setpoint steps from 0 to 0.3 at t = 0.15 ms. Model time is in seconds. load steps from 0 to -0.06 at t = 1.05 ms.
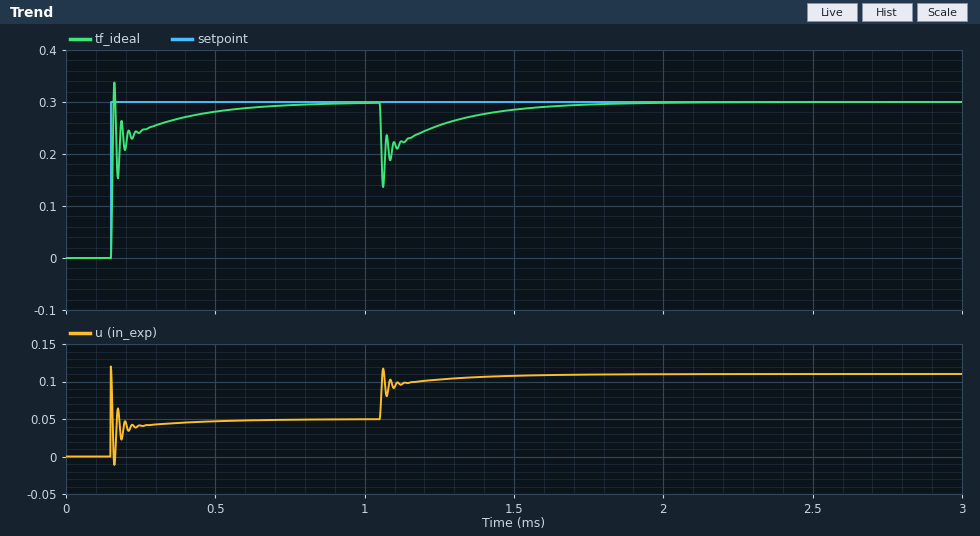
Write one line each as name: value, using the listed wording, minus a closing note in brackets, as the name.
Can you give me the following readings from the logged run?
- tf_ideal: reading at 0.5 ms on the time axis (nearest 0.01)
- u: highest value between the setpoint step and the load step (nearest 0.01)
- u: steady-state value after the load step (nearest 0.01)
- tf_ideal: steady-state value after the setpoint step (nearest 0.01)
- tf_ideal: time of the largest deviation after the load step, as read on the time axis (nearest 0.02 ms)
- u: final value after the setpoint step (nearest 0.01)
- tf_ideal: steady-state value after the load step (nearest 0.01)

tf_ideal: reading at 0.5 ms on the time axis: 0.28
u: highest value between the setpoint step and the load step: 0.12
u: steady-state value after the load step: 0.11
tf_ideal: steady-state value after the setpoint step: 0.30
tf_ideal: time of the largest deviation after the load step, as read on the time axis: 1.06 ms
u: final value after the setpoint step: 0.05
tf_ideal: steady-state value after the load step: 0.30
